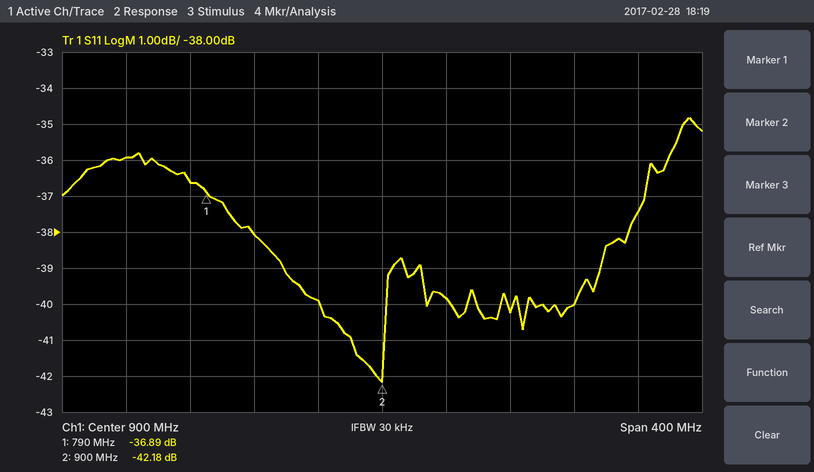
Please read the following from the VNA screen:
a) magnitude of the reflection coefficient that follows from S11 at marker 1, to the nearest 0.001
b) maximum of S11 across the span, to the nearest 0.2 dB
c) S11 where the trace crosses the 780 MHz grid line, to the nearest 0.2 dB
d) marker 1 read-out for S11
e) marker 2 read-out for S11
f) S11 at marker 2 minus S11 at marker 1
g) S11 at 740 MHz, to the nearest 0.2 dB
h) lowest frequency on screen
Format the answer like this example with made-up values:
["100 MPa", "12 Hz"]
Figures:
["0.014", "-34.8 dB", "-36.6 dB", "-36.89 dB", "-42.18 dB", "-5.29 dB", "-36.0 dB", "700 MHz"]
